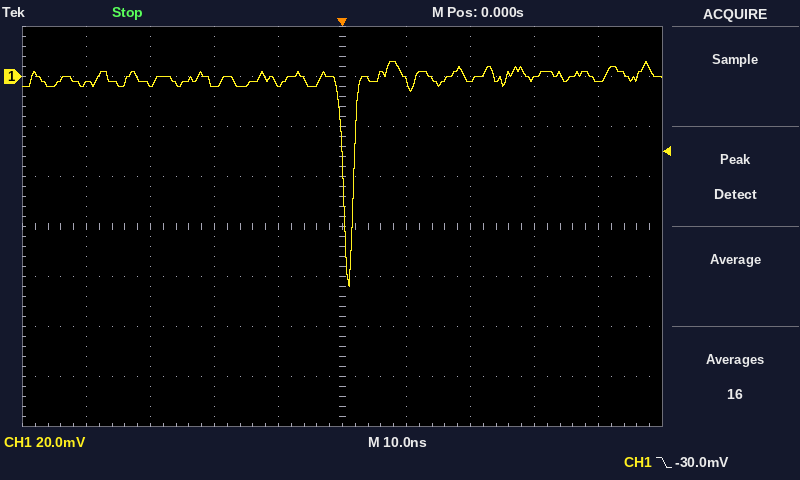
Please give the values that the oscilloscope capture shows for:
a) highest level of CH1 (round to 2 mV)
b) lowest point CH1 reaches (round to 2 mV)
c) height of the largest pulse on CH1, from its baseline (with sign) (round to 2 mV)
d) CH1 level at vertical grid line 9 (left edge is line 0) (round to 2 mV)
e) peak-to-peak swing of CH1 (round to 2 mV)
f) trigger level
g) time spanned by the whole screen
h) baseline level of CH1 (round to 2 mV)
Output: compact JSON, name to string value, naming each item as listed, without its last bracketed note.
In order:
{"highest level of CH1": "6 mV", "lowest point CH1 reaches": "-84 mV", "height of the largest pulse on CH1, from its baseline (with sign)": "-84 mV", "CH1 level at vertical grid line 9 (left edge is line 0)": "-2 mV", "peak-to-peak swing of CH1": "90 mV", "trigger level": "-30.0 mV", "time spanned by the whole screen": "100 ns", "baseline level of CH1": "0 mV"}
